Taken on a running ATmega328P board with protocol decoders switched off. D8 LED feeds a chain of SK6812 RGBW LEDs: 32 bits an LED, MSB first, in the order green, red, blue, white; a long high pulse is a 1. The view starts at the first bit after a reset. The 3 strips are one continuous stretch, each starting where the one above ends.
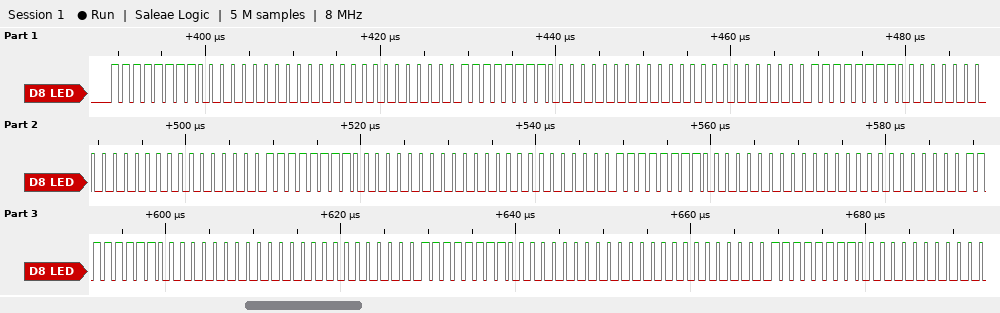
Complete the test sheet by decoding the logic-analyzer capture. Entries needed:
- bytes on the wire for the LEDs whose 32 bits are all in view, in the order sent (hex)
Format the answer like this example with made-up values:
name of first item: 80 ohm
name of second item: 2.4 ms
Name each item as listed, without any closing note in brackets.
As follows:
bytes on the wire for the LEDs whose 32 bits are all in view, in the order sent: FF 00 00 00 FF 00 00 00 FF 00 00 00 FF 00 00 00 FF 00 00 00 FF 00 00 00 FF 00 00 00
